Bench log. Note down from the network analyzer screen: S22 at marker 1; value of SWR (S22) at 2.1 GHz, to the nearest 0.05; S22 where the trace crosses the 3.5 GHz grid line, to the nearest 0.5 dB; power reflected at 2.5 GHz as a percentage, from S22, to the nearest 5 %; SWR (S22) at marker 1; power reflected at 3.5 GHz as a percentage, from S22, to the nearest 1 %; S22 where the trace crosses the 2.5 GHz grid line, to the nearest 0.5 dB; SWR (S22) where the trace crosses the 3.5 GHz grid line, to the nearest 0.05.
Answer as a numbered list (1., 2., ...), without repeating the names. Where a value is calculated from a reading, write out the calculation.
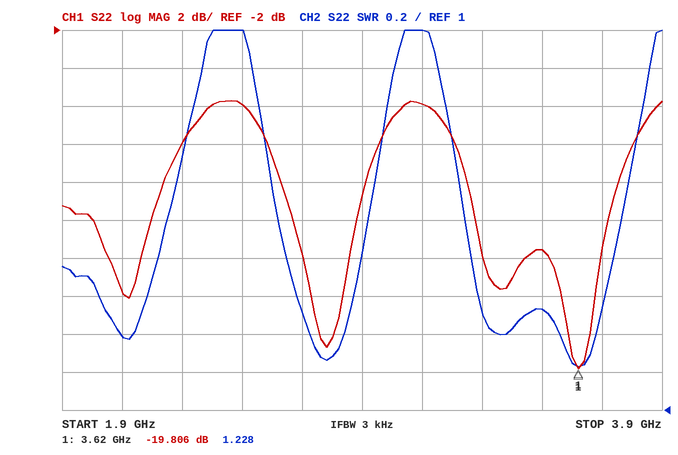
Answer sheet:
1. -19.806 dB
2. 1.40
3. -13.5 dB
4. 10^(-6/10) ≈ 25 %
5. 1.228
6. 10^(-13.5/10) ≈ 4 %
7. -6.0 dB
8. 1.55
